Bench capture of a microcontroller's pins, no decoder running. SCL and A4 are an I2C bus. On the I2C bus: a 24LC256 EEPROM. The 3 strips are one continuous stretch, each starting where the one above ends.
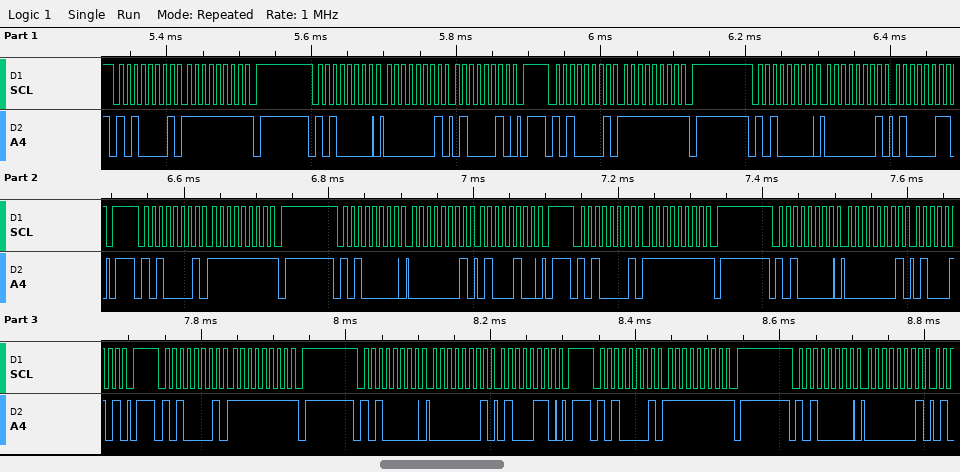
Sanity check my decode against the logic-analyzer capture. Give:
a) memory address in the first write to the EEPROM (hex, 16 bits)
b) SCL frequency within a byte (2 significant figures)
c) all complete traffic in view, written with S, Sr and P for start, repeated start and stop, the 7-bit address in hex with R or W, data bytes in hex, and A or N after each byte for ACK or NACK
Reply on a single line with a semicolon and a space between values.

0x0142; 100 kHz; S 50R A FF N P S 50W A 01 A 42 A P S 50R A FF N P S 50W A 01 A 43 A P S 50R A FF N P S 50W A 01 A 44 A P S 50R A FF N P S 50W A 01 A 45 A P S 50R A FF N P S 50W A 01 A 46 A P S 50R A FF N P S 50W A 01 A
